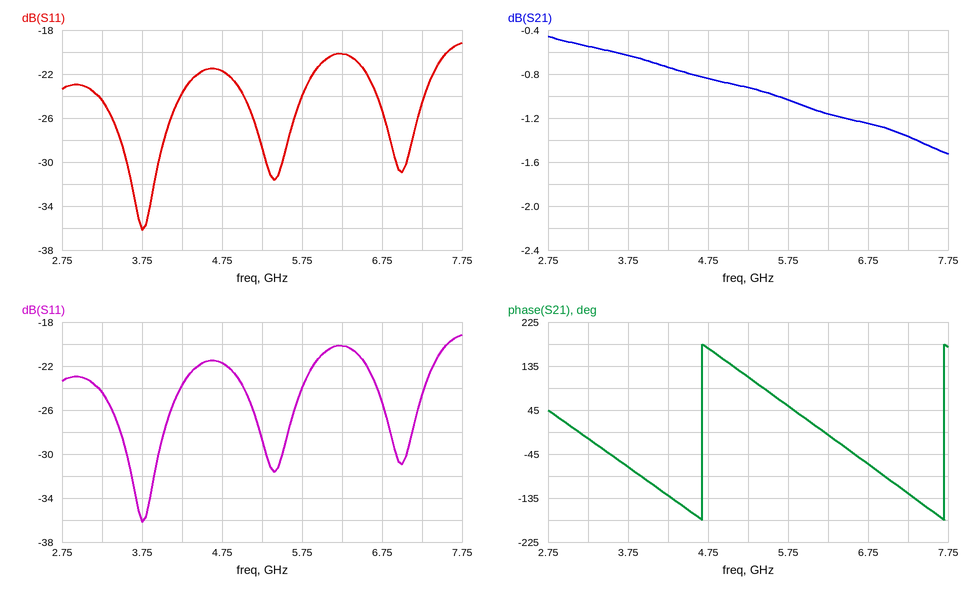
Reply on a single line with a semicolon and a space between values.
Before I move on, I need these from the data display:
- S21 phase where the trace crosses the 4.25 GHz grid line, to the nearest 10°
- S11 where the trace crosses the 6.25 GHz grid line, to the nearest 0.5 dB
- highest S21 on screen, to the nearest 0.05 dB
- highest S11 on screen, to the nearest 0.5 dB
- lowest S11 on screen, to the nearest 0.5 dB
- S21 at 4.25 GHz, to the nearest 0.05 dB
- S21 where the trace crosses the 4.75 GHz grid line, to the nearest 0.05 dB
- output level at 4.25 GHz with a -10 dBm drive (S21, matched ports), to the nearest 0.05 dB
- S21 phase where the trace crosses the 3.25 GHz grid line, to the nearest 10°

-130°; -20.0 dB; -0.45 dB; -19.0 dB; -36.0 dB; -0.75 dB; -0.85 dB; -10.75 dBm; -10°
